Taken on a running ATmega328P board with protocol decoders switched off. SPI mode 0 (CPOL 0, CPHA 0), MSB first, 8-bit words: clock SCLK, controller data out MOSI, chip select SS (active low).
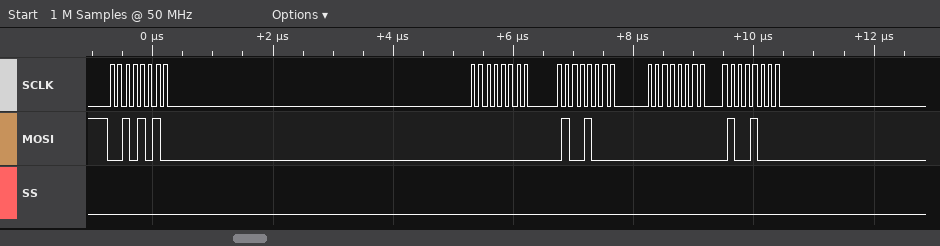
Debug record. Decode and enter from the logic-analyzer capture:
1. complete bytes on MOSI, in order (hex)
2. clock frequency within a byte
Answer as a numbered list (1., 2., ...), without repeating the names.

1. 2A 00 48 00 48
2. 8 MHz
